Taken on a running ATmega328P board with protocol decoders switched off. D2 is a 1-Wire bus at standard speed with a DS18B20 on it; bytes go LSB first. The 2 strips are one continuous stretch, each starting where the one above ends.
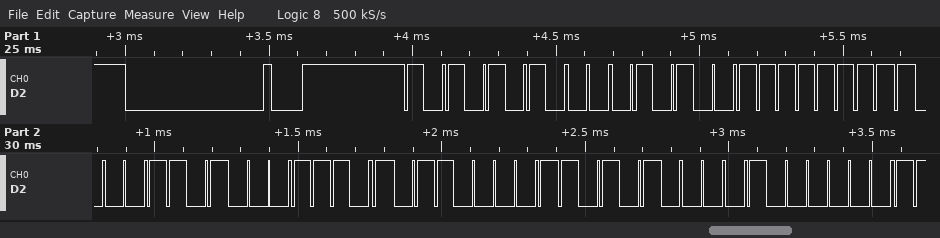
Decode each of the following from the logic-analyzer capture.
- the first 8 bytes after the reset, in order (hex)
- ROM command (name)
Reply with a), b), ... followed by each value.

a) 55 28 FF B1 B8 86 15 02
b) Match ROM
